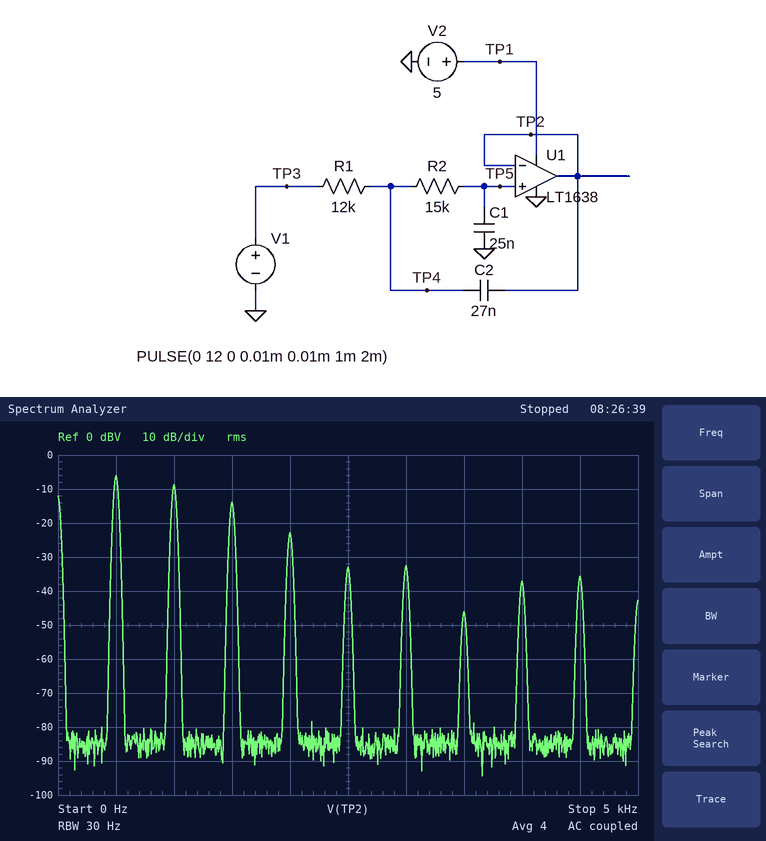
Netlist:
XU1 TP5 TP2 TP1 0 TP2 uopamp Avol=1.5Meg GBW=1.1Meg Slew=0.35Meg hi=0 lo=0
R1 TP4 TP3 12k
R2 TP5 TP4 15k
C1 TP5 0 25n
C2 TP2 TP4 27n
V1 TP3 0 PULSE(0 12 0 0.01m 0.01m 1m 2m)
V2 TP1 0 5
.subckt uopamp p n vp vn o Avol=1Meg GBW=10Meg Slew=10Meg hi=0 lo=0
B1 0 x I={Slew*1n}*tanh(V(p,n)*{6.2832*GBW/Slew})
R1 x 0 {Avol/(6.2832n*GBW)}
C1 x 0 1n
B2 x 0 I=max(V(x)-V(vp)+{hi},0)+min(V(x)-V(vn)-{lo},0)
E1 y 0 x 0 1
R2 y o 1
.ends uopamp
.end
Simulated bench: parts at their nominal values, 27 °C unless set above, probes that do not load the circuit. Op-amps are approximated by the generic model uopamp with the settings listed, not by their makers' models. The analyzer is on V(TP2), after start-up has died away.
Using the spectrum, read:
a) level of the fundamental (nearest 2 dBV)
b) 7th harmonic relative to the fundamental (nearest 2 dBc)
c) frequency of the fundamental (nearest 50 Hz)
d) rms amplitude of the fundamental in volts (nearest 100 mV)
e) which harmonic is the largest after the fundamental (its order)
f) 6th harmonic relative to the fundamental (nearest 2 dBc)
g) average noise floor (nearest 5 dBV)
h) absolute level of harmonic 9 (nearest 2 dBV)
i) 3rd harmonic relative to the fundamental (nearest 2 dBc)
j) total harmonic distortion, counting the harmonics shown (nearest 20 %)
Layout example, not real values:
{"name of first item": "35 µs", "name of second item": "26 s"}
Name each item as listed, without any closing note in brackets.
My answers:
{"level of the fundamental": "-6 dBV", "7th harmonic relative to the fundamental": "-40 dBc", "frequency of the fundamental": "500 Hz", "rms amplitude of the fundamental in volts": "500 mV", "which harmonic is the largest after the fundamental": "2", "6th harmonic relative to the fundamental": "-26 dBc", "average noise floor": "-85 dBV", "absolute level of harmonic 9": "-36 dBV", "3rd harmonic relative to the fundamental": "-8 dBc", "total harmonic distortion, counting the harmonics shown": "80 %"}
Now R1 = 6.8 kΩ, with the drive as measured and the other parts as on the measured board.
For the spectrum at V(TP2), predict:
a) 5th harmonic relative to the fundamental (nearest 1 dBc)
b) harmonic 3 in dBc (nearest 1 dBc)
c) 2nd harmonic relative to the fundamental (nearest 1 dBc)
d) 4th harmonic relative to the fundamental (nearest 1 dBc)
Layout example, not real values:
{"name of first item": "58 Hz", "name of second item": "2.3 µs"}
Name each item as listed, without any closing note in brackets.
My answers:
{"5th harmonic relative to the fundamental": "-21 dBc", "harmonic 3 in dBc": "-11 dBc", "2nd harmonic relative to the fundamental": "-4 dBc", "4th harmonic relative to the fundamental": "-20 dBc"}
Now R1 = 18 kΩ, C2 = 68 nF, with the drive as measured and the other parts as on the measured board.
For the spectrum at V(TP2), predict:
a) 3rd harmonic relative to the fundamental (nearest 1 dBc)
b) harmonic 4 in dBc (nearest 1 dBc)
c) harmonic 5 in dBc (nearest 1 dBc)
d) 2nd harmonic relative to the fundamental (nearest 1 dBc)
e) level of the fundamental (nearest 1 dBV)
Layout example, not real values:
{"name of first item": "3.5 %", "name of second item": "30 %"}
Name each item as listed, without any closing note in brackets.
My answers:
{"3rd harmonic relative to the fundamental": "0 dBc", "harmonic 4 in dBc": "0 dBc", "harmonic 5 in dBc": "-1 dBc", "2nd harmonic relative to the fundamental": "0 dBc", "level of the fundamental": "-51 dBV"}
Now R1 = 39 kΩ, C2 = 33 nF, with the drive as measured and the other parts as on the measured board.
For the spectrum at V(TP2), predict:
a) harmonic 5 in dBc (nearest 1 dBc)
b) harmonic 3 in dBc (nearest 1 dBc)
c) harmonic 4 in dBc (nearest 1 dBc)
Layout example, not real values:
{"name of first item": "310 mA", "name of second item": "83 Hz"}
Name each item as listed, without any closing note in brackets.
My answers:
{"harmonic 5 in dBc": "-11 dBc", "harmonic 3 in dBc": "-7 dBc", "harmonic 4 in dBc": "-33 dBc"}
